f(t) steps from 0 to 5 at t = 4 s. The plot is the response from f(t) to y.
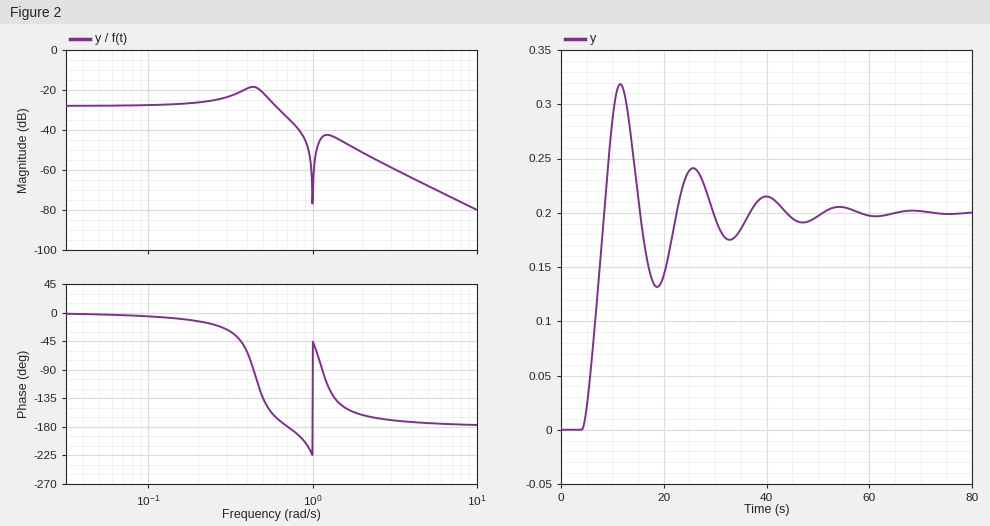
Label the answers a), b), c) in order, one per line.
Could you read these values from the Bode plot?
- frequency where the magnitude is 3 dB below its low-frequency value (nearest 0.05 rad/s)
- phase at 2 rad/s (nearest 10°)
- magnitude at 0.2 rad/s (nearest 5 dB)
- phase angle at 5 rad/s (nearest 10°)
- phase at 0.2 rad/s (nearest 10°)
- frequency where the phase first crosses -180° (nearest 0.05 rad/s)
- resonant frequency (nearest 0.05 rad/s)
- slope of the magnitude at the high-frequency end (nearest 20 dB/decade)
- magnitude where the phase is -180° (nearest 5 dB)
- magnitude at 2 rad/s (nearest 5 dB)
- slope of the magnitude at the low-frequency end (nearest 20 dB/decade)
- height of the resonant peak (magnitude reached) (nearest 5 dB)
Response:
a) 0.65 rad/s
b) -160°
c) -25 dB
d) -170°
e) -10°
f) 0.70 rad/s
g) 0.45 rad/s
h) -40 dB/decade
i) -35 dB
j) -50 dB
k) 0 dB/decade
l) -20 dB
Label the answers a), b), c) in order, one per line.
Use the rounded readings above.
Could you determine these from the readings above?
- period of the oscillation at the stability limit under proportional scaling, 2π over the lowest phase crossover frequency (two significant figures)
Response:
a) 9.0 s
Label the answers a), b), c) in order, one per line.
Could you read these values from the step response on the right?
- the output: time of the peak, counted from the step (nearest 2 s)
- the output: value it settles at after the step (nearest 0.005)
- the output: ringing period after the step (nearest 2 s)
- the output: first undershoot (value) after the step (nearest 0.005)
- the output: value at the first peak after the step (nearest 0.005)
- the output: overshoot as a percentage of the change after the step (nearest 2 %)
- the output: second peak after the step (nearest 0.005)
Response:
a) 8 s
b) 0.200
c) 14 s
d) 0.130
e) 0.320
f) 60 %
g) 0.240
